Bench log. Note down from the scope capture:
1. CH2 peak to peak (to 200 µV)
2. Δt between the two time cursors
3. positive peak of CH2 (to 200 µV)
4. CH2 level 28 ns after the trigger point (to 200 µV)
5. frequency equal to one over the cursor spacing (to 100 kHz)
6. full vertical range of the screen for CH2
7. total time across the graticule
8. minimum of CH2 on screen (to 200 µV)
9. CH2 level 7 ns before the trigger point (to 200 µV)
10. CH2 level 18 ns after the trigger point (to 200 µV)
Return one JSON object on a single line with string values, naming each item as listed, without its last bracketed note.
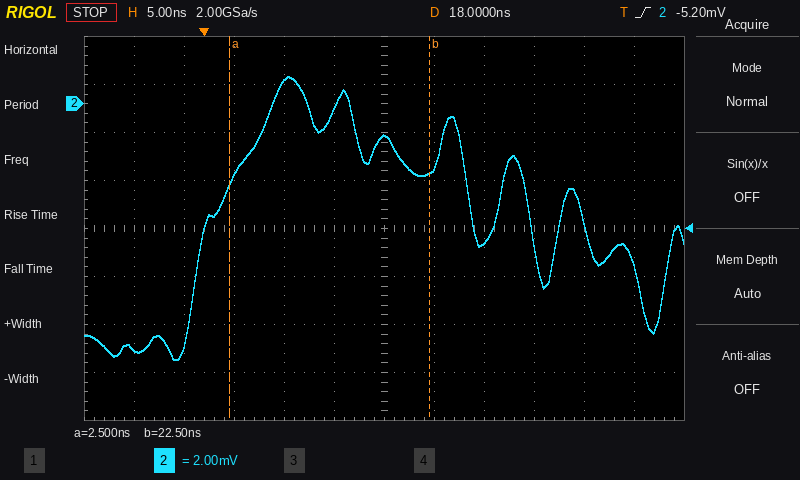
{"CH2 peak to peak": "11.8 mV", "Δt between the two time cursors": "20.0 ns", "positive peak of CH2": "1.2 mV", "CH2 level 28 ns after the trigger point": "-5.8 mV", "frequency equal to one over the cursor spacing": "50.0 MHz", "full vertical range of the screen for CH2": "16 mV", "total time across the graticule": "60 ns", "minimum of CH2 on screen": "-10.6 mV", "CH2 level 7 ns before the trigger point": "-10.2 mV", "CH2 level 18 ns after the trigger point": "-1.4 mV"}
